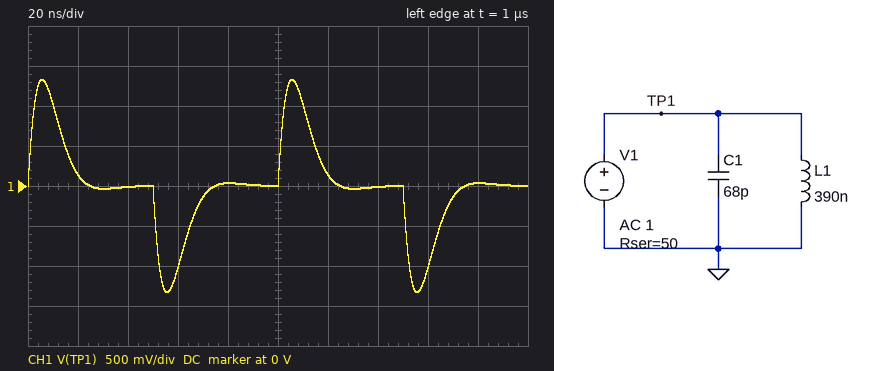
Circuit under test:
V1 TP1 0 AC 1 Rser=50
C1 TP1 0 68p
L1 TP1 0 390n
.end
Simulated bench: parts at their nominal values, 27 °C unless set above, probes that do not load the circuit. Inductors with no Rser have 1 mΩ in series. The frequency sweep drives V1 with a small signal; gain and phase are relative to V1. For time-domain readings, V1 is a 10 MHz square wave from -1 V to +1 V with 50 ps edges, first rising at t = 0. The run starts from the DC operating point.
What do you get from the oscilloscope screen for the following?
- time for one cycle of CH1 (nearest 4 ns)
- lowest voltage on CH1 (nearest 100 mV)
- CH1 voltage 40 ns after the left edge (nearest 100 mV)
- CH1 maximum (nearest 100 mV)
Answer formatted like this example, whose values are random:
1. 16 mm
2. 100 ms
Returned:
1. 100 ns
2. -1.3 V
3. 0 V
4. 1.3 V
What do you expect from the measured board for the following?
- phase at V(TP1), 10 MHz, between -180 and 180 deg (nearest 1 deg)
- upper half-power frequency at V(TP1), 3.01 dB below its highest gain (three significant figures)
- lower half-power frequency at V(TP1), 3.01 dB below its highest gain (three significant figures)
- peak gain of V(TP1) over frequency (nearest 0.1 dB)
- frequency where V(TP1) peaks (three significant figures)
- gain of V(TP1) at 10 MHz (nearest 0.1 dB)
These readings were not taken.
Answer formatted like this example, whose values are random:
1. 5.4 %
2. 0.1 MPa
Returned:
1. 61 deg
2. 62.2 MHz
3. 15.4 MHz
4. 0 dB
5. 30.9 MHz
6. -6.4 dB
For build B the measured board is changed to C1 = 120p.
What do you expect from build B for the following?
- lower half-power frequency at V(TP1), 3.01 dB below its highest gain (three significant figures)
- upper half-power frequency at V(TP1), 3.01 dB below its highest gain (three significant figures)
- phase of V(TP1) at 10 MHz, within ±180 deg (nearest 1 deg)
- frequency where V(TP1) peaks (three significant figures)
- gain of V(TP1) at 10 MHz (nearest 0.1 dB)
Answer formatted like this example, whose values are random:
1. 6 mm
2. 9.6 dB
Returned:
1. 13.5 MHz
2. 40.0 MHz
3. 59 deg
4. 23.3 MHz
5. -5.8 dB
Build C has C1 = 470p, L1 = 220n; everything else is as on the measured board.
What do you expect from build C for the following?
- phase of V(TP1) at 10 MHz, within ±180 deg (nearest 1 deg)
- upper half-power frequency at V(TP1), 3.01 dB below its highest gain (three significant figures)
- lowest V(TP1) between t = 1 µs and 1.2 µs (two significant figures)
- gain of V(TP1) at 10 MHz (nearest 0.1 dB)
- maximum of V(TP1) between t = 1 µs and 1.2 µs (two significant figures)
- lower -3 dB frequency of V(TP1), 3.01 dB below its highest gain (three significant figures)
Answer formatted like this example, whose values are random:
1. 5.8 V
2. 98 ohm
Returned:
1. 65 deg
2. 19.4 MHz
3. -630 mV
4. -7.5 dB
5. 630 mV
6. 12.6 MHz
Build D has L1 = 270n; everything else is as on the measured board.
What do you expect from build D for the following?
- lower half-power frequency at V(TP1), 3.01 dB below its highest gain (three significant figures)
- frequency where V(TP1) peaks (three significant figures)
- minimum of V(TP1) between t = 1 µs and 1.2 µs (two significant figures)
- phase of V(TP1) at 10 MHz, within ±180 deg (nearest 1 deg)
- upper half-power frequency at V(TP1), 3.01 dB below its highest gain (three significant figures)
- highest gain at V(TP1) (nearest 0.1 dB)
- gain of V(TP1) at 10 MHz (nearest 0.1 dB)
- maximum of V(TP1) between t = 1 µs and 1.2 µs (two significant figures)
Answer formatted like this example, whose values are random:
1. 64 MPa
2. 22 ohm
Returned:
1. 20.5 MHz
2. 37.1 MHz
3. -1.2 V
4. 70 deg
5. 67.3 MHz
6. 0 dB
7. -9.3 dB
8. 1.2 V
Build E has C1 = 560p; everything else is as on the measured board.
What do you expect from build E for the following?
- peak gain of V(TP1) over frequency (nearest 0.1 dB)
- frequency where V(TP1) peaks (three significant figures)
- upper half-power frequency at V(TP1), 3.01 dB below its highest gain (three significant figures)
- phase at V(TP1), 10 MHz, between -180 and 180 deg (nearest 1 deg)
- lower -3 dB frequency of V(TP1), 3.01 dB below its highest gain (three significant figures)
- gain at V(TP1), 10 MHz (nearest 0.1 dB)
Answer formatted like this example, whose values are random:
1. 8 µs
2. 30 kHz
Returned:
1. 0 dB
2. 10.8 MHz
3. 14.0 MHz
4. 16 deg
5. 8.30 MHz
6. -0.3 dB
